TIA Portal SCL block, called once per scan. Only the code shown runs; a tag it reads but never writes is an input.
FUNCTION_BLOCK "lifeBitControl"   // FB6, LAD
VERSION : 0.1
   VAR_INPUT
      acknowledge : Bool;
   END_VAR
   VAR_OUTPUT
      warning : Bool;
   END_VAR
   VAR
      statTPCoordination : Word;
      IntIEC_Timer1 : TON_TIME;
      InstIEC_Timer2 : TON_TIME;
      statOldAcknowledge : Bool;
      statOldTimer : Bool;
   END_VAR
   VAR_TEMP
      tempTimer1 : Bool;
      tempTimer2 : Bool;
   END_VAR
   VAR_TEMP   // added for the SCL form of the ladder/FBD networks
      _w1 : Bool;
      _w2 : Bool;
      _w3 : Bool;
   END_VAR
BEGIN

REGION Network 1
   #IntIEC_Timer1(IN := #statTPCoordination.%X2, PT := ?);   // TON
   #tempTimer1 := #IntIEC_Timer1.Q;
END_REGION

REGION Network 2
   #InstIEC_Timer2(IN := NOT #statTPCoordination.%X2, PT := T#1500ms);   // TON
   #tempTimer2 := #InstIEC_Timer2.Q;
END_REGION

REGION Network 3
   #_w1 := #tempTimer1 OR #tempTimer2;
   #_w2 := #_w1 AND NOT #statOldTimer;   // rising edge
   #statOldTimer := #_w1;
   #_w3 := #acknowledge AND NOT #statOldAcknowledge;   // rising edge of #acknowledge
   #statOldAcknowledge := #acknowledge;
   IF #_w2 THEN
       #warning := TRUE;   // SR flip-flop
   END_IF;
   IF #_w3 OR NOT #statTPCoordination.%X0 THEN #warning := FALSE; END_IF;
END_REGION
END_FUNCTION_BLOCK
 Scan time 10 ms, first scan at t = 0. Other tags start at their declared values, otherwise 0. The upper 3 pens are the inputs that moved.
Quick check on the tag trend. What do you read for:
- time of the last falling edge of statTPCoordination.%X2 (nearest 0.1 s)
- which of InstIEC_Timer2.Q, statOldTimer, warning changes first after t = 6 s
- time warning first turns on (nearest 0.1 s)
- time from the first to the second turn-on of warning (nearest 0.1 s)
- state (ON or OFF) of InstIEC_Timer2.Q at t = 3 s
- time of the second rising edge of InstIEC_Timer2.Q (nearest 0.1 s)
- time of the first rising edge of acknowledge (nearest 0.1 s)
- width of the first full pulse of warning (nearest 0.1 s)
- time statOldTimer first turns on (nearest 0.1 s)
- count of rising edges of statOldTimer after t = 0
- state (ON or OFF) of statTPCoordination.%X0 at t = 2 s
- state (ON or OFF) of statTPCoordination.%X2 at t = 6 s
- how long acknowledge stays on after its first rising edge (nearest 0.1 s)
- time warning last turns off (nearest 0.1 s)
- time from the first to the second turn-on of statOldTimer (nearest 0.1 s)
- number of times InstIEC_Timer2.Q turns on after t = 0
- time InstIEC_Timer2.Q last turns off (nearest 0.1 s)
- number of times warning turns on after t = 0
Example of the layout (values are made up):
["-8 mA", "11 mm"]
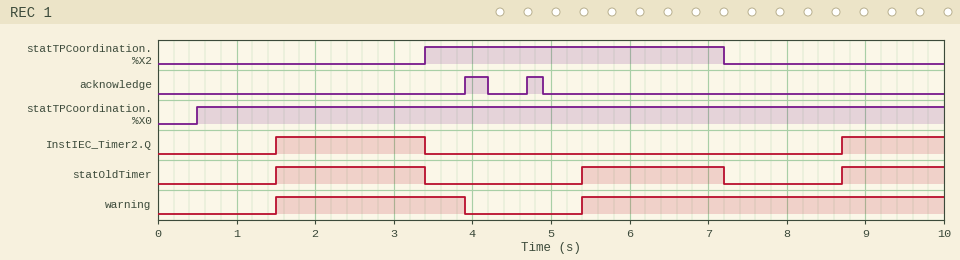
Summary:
["7.2 s", "statOldTimer", "1.5 s", "3.9 s", "ON", "8.7 s", "3.9 s", "2.4 s", "1.5 s", "3", "ON", "ON", "0.3 s", "3.9 s", "3.9 s", "2", "3.4 s", "2"]
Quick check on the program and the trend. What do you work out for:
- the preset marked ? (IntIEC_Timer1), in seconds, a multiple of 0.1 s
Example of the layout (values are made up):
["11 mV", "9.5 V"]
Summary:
["2.0 s"]
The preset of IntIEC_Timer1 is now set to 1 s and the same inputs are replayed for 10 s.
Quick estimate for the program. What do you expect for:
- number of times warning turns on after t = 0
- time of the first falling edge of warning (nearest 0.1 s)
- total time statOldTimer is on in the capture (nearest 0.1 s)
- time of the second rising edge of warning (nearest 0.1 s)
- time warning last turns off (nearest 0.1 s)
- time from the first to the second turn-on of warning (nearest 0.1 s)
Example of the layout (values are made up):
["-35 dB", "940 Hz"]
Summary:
["3", "3.9 s", "6.0 s", "4.4 s", "4.7 s", "2.9 s"]
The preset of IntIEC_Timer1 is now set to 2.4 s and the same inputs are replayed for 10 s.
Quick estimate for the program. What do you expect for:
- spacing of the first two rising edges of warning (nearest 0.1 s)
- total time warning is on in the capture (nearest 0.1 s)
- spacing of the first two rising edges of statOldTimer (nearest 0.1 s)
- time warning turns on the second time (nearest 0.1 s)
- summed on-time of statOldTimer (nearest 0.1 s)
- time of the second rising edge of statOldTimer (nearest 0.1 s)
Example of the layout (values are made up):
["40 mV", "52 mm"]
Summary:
["4.3 s", "6.6 s", "4.3 s", "5.8 s", "4.6 s", "5.8 s"]
